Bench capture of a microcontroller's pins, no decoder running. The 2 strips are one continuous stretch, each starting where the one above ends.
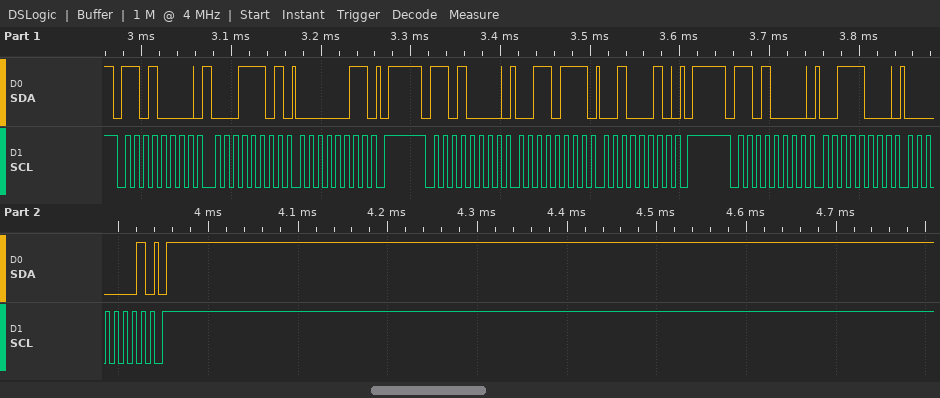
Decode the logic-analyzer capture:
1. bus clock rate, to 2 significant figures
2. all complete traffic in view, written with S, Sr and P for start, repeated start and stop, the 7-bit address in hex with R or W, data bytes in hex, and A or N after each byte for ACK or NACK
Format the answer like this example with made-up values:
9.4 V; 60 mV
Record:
100 kHz; S 68W A 1D A 03 A P S 68W A 37 A 22 A P S 68W A 38 A 01 A P
